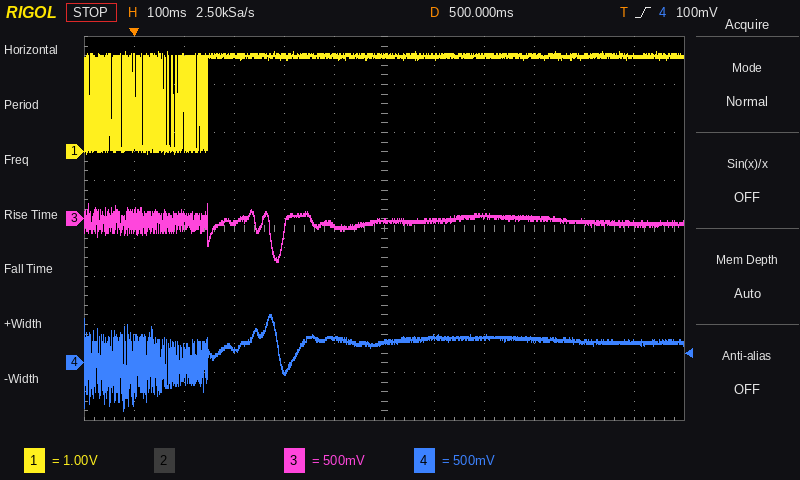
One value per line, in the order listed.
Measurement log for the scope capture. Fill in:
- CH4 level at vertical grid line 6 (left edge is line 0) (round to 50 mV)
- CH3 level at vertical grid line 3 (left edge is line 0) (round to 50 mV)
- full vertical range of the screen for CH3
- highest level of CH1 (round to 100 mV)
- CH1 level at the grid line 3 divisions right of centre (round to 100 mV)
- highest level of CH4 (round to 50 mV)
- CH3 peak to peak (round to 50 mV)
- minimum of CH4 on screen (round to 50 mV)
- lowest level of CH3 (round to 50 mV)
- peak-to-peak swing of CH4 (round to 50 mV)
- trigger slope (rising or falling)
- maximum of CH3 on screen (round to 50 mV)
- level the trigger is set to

200 mV
-50 mV
4 V
2.1 V
2.0 V
500 mV
600 mV
-500 mV
-450 mV
1.00 V
rising
150 mV
100 mV
